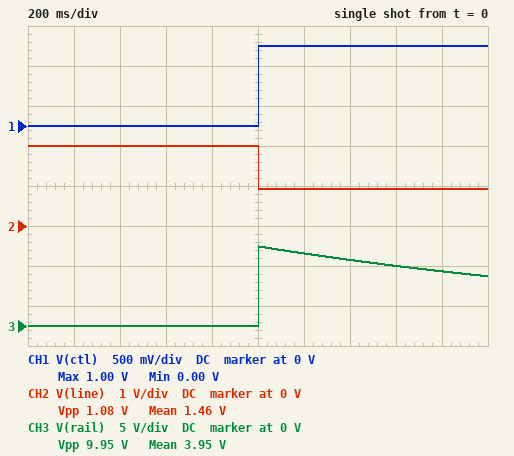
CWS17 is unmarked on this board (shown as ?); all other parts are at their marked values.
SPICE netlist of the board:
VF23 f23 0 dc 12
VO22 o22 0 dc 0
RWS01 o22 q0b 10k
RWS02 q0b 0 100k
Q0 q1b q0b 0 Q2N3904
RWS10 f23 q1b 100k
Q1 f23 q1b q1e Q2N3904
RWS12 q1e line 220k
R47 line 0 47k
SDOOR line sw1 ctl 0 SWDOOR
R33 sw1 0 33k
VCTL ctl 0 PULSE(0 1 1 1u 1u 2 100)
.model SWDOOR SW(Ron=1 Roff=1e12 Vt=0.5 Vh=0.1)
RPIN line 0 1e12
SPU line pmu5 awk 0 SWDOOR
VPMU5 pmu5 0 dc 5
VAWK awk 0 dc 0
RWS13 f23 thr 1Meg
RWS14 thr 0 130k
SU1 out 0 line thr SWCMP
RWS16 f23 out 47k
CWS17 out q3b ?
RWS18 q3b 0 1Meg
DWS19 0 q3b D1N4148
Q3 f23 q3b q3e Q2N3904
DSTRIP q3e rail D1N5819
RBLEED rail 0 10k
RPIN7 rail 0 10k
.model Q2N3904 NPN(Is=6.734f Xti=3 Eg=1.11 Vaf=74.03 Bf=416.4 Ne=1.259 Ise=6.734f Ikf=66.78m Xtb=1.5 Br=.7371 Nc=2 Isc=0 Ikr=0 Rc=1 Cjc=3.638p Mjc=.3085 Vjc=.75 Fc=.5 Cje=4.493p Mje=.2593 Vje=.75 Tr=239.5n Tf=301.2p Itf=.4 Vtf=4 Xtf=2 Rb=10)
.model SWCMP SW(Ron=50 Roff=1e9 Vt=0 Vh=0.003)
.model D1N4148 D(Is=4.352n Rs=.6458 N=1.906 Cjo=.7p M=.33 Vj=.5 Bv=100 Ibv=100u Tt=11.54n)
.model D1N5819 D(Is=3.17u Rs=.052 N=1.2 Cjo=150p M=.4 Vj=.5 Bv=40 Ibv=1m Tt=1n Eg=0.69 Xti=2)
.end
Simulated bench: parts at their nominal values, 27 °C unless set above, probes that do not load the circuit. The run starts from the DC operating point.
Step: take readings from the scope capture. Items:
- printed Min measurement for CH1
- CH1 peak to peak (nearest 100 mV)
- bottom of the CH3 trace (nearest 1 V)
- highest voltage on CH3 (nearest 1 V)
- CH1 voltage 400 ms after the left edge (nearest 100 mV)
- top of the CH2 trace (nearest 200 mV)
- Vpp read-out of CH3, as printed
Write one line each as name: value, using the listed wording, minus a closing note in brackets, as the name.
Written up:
printed Min measurement for CH1: 0.00 V
CH1 peak to peak: 1.0 V
bottom of the CH3 trace: 0 V
highest voltage on CH3: 10 V
CH1 voltage 400 ms after the left edge: 0 V
top of the CH2 trace: 2.0 V
Vpp read-out of CH3, as printed: 9.95 V
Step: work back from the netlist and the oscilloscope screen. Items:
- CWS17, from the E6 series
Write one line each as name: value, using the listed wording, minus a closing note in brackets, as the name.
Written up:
CWS17, from the E6 series: 4.7 µF
